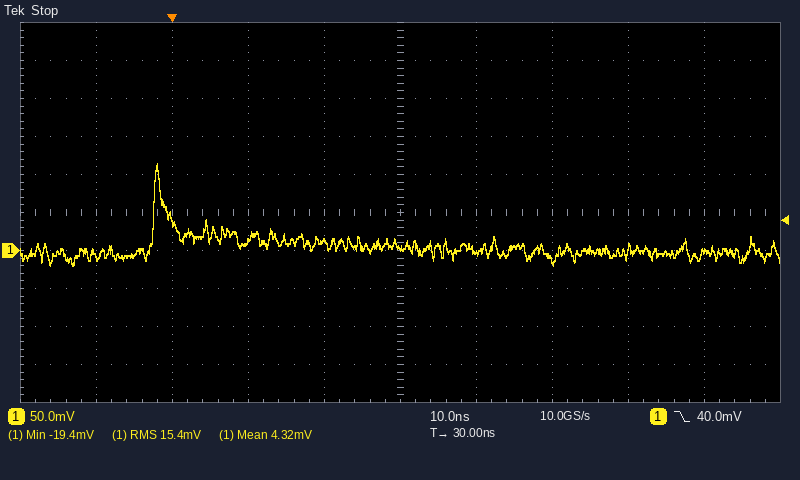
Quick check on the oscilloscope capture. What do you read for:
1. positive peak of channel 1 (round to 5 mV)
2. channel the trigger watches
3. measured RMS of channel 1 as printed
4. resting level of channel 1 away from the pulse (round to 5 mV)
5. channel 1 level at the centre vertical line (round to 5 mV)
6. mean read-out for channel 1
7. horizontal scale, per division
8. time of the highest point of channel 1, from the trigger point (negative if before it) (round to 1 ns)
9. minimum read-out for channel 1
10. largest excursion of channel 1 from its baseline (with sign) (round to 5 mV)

115 mV
channel 1
15.4 mV
0 mV
5 mV
4.32 mV
10 ns
-2 ns
-19.4 mV
+115 mV
